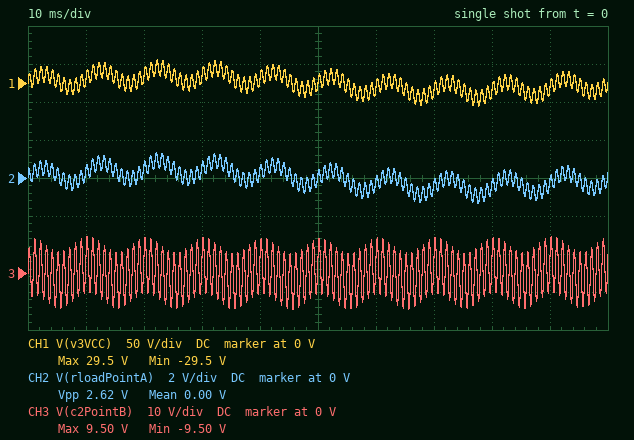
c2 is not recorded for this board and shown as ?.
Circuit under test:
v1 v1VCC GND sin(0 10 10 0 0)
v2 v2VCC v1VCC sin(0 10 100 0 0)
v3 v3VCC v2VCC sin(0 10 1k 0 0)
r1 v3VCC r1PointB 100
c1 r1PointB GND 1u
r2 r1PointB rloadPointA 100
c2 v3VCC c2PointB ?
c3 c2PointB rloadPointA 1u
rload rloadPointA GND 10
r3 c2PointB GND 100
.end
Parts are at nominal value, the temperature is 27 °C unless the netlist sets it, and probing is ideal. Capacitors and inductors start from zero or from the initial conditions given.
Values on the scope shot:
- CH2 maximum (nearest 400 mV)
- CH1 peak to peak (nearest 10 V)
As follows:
1.2 V
60 V
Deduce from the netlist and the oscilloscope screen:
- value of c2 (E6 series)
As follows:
3.3 µF
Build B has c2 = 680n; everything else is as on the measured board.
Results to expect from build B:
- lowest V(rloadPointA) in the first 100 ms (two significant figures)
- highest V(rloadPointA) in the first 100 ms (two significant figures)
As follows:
-1.2 V
1.2 V
